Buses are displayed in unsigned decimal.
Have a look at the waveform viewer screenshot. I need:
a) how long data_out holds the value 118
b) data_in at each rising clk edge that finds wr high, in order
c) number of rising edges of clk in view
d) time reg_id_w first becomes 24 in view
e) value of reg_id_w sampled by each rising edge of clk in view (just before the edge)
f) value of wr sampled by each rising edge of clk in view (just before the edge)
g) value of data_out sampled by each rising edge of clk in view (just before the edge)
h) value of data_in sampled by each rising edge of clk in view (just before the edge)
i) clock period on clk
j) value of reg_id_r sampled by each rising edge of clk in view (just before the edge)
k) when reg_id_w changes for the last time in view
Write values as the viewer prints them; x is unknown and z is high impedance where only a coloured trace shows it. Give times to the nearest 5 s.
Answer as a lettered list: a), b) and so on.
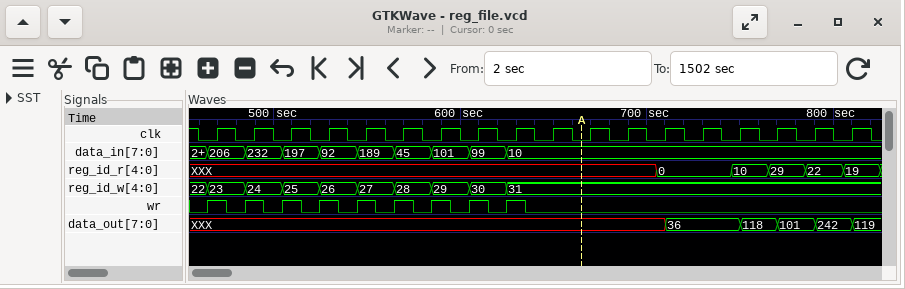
a) 20 s
b) 206, 232, 197, 92, 189, 45, 101, 99, 10
c) 18
d) 485 s
e) 23, 24, 25, 26, 27, 28, 29, 30, 31, 31, 31, 31, 31, 31, 31, 31, 31, 31
f) 1 1 1 1 1 1 1 1 1 0 0 0 0 0 0 0 0 0
g) XXX, XXX, XXX, XXX, XXX, XXX, XXX, XXX, XXX, XXX, XXX, XXX, XXX, 36, 36, 118, 101, 242
h) 206, 232, 197, 92, 189, 45, 101, 99, 10, 10, 10, 10, 10, 10, 10, 10, 10, 10
i) 20 s
j) XXX, XXX, XXX, XXX, XXX, XXX, XXX, XXX, XXX, XXX, XXX, XXX, 0, 0, 10, 29, 22, 19
k) 625 s
